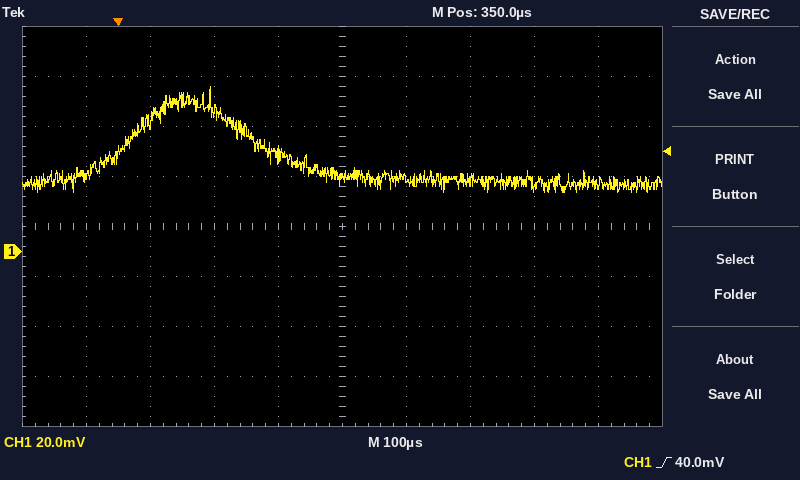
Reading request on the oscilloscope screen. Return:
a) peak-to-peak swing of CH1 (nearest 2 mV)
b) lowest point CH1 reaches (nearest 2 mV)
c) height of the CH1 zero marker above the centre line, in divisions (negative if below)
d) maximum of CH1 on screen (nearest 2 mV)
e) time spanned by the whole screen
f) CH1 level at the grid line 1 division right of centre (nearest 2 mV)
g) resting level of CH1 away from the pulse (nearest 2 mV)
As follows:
42 mV
24 mV
-0.5 div
66 mV
1 ms
30 mV
28 mV
